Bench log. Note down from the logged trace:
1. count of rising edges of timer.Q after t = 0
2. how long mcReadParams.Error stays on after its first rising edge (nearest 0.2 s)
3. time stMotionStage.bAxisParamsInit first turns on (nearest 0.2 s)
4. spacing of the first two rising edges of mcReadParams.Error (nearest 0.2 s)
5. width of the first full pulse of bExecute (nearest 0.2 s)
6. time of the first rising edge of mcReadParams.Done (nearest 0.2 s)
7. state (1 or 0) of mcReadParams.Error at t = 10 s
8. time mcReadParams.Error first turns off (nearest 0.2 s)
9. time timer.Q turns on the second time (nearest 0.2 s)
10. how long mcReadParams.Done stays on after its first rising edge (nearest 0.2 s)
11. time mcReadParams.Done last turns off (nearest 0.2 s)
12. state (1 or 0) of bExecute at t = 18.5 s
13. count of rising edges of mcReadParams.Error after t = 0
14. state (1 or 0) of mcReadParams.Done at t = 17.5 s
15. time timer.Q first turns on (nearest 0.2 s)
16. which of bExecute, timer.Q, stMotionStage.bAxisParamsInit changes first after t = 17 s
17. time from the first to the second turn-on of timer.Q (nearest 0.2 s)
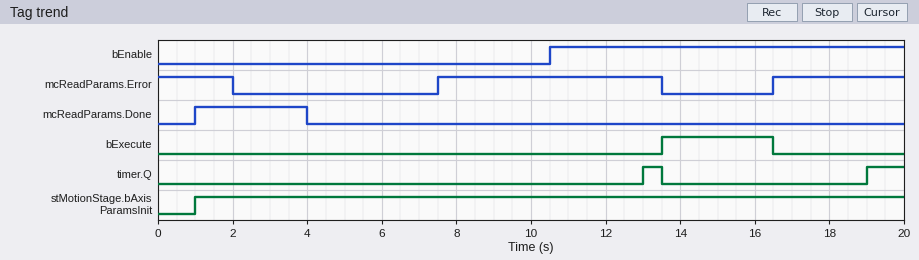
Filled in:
2
6.0 s
1.0 s
9.0 s
3.0 s
1.0 s
1
2.0 s
19.0 s
3.0 s
4.0 s
0
2
0
13.0 s
timer.Q
6.0 s
